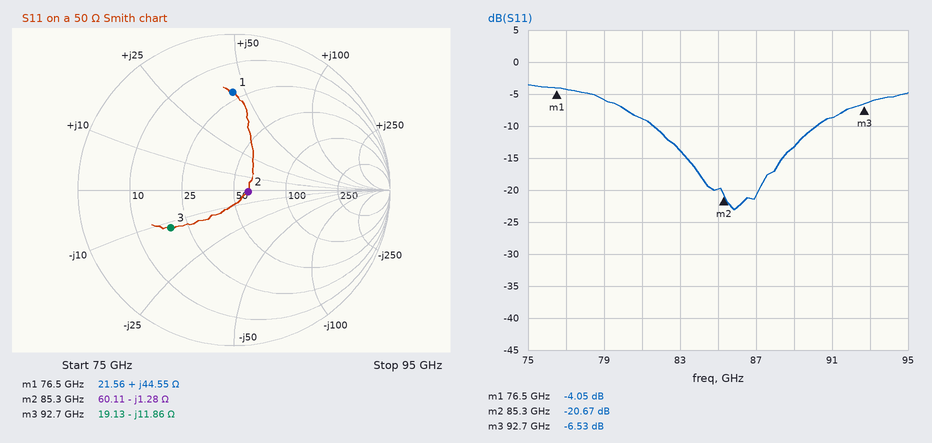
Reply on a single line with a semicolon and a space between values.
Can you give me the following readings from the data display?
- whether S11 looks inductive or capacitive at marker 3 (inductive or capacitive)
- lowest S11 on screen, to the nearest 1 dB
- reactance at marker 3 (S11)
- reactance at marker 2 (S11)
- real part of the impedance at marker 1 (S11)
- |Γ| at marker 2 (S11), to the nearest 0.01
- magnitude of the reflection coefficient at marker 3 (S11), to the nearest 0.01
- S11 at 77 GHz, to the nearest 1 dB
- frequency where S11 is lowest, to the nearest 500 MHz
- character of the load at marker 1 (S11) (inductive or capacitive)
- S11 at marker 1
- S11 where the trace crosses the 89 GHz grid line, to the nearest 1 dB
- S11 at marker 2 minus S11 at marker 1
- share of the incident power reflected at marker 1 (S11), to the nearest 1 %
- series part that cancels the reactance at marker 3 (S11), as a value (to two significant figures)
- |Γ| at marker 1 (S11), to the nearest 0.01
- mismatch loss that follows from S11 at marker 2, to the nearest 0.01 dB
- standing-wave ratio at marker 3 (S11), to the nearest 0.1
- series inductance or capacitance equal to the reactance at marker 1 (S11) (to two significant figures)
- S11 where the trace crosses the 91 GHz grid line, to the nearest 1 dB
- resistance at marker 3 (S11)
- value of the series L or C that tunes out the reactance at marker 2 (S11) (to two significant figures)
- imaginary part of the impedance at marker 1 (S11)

capacitive; -23 dB; -11.86 Ω; -1.28 Ω; 21.56 Ω; 0.09; 0.47; -4 dB; 86.0 GHz; inductive; -4.05 dB; -13 dB; -16.62 dB; 39 %; 20 pH; 0.63; 0.04 dB; 2.8; 93 pH; -9 dB; 19.13 Ω; 2.4 pH; +44.55 Ω
